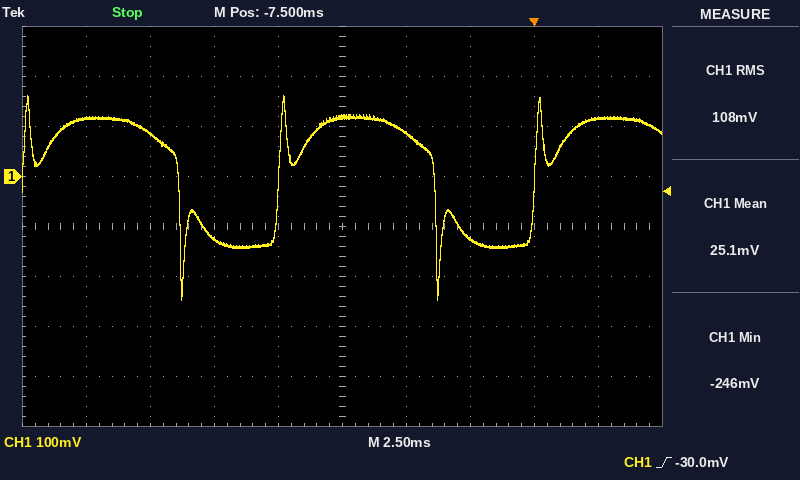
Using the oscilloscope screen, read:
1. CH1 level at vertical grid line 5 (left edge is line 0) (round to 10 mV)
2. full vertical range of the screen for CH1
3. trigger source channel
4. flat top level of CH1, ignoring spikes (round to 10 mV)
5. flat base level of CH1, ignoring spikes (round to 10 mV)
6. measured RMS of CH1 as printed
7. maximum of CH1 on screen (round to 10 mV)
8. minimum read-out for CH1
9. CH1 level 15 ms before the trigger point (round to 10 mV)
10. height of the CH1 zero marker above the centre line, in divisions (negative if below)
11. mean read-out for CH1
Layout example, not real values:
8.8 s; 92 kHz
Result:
120 mV; 800 mV; CH1; 120 mV; -140 mV; 108 mV; 160 mV; -246 mV; 90 mV; +1.0 div; 25.1 mV
